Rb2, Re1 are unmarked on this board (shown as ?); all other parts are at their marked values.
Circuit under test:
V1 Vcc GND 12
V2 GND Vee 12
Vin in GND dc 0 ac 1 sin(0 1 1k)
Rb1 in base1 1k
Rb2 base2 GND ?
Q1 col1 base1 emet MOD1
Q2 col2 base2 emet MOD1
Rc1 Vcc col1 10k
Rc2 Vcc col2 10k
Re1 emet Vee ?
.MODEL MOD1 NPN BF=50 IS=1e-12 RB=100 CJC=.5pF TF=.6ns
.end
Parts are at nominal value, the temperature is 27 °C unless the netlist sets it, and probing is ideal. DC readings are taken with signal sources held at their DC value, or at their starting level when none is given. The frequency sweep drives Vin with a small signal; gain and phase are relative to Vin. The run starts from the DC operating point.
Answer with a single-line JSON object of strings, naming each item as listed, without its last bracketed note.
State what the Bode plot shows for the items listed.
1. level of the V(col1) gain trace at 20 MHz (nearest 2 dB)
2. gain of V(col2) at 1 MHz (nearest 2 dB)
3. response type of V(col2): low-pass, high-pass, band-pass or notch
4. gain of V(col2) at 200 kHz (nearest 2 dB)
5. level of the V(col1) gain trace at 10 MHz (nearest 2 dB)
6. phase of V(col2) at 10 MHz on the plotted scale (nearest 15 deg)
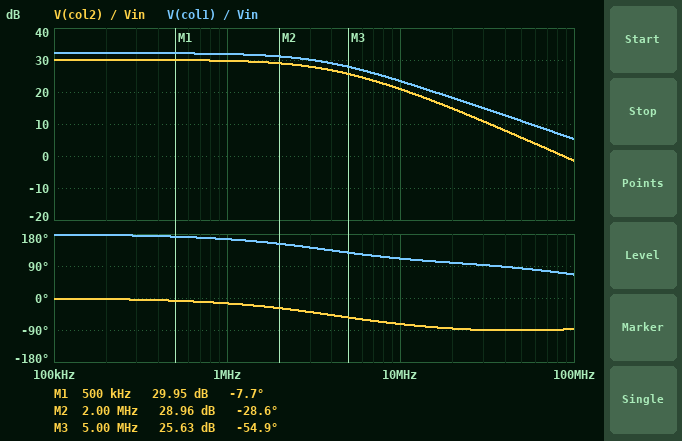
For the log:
{"level of the V(col1) gain trace at 20 MHz": "18 dB", "gain of V(col2) at 1 MHz": "30 dB", "response type of V(col2): low-pass, high-pass, band-pass or notch": "low-pass", "gain of V(col2) at 200 kHz": "30 dB", "level of the V(col1) gain trace at 10 MHz": "24 dB", "phase of V(col2) at 10 MHz on the plotted scale": "-75 deg"}
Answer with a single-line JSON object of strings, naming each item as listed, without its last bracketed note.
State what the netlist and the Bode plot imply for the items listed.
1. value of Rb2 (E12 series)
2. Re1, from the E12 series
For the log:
{"value of Rb2": "820 Ω", "Re1, from the E12 series": "4.7 kΩ"}
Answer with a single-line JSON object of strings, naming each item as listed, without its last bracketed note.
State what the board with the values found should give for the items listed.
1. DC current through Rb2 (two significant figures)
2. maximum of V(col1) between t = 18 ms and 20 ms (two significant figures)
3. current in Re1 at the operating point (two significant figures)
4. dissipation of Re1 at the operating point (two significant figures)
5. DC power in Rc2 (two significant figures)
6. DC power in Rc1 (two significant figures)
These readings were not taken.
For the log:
{"DC current through Rb2": "25 µA", "maximum of V(col1) between t = 18 ms and 20 ms": "12 V", "current in Re1 at the operating point": "2.4 mA", "dissipation of Re1 at the operating point": "28 mW", "DC power in Rc2": "15 mW", "DC power in Rc1": "13 mW"}
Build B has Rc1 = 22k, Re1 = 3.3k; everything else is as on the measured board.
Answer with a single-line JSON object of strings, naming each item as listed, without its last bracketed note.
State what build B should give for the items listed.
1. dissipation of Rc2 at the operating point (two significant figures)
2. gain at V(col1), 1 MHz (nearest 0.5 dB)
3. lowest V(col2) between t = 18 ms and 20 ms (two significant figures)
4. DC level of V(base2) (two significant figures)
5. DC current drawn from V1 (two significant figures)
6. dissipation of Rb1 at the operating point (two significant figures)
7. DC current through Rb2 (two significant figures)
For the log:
{"dissipation of Rc2 at the operating point": "17 mW", "gain at V(col1), 1 MHz": "-9.0 dB", "lowest V(col2) between t = 18 ms and 20 ms": "-1.6 V", "DC level of V(base2)": "-600 mV", "DC current drawn from V1": "1.9 mA", "dissipation of Rb1 at the operating point": "380 µW", "DC current through Rb2": "730 µA"}
